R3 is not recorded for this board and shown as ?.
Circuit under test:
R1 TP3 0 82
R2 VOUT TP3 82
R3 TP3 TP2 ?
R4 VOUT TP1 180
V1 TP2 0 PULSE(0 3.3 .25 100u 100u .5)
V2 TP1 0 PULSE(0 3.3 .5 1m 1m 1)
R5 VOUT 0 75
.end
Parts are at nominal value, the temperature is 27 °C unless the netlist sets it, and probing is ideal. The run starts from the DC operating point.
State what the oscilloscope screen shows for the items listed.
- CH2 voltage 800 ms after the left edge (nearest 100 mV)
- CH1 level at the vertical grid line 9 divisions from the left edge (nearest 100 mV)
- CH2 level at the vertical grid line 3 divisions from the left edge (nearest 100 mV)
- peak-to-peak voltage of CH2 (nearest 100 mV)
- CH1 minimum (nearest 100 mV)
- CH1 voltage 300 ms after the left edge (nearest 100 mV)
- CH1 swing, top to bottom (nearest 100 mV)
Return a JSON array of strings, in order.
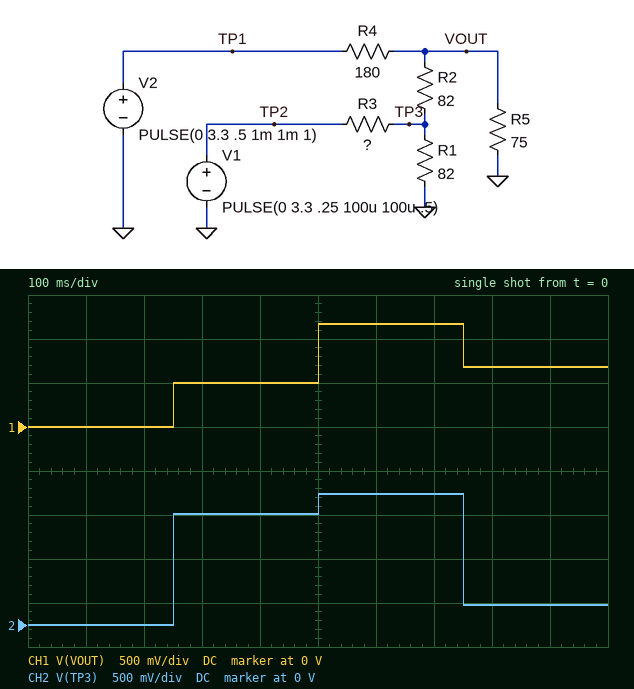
["200 mV", "700 mV", "1.3 V", "1.5 V", "0 V", "500 mV", "1.2 V"]
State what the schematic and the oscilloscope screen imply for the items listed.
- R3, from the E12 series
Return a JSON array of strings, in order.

["82 Ω"]
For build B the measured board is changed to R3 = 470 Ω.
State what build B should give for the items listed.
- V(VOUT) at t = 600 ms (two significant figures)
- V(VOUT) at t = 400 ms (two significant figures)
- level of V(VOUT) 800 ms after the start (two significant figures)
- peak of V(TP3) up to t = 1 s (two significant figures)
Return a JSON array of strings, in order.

["850 mV", "130 mV", "720 mV", "650 mV"]
